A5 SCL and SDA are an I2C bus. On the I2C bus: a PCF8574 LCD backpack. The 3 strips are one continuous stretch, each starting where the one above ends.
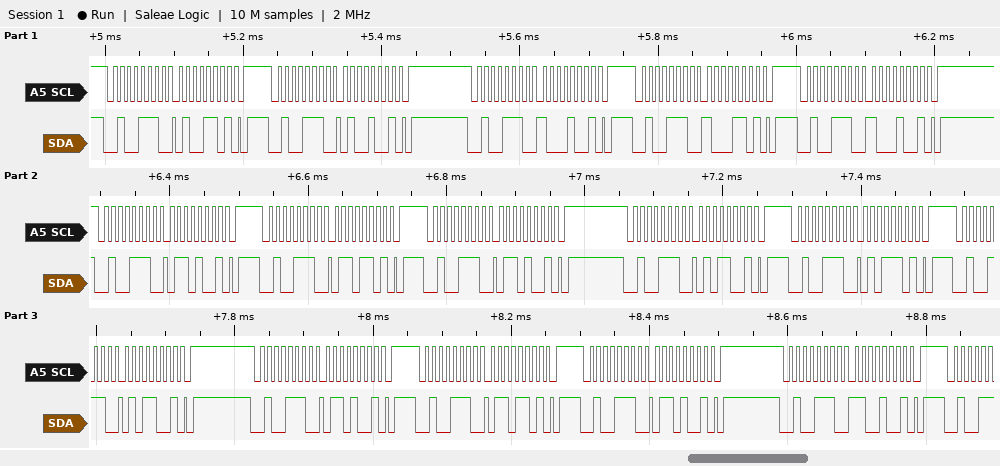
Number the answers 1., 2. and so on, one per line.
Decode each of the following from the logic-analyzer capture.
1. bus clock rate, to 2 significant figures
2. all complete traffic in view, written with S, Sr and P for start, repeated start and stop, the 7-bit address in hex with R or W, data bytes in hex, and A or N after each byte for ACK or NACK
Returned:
1. 100 kHz
2. S 27W A 4D A P S 27W A 49 A P S 27W A 89 A P S 27W A 8D A P S 27W A 89 A P S 27W A 69 A P S 27W A 6D A P S 27W A 69 A P S 27W A 59 A P S 27W A 5D A P S 27W A 59 A P S 27W A 69 A P S 27W A 6D A P S 27W A 69 A P S 27W A C9 A P
